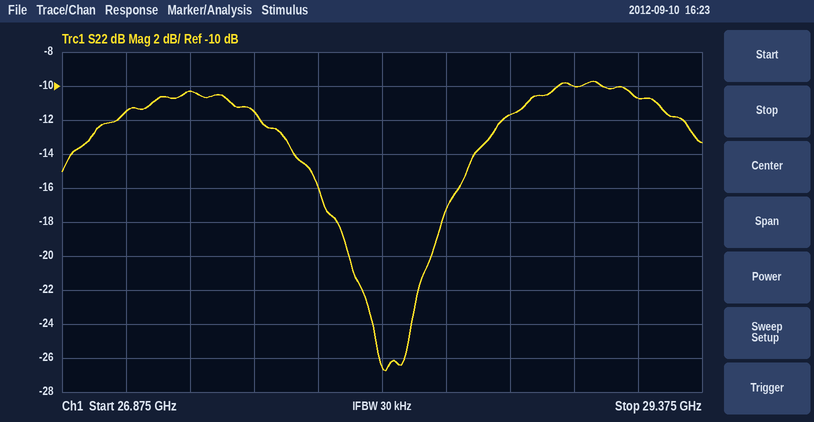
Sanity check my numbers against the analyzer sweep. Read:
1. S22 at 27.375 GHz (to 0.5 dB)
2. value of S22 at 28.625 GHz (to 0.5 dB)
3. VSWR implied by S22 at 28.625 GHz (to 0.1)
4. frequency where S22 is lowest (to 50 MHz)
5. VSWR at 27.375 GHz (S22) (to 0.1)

-10.5 dB
-11.5 dB
1.7
28.15 GHz
1.9
